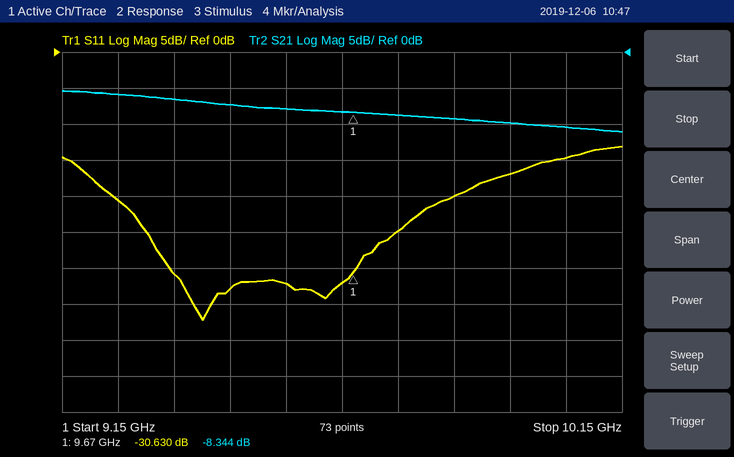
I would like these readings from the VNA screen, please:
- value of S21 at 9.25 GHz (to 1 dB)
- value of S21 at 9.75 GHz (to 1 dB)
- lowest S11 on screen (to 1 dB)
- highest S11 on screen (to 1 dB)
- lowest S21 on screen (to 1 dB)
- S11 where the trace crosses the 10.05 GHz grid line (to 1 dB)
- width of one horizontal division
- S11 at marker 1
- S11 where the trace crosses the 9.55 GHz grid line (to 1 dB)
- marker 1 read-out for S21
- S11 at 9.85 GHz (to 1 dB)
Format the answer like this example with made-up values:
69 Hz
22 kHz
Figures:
-6 dB
-9 dB
-37 dB
-13 dB
-11 dB
-15 dB
100 MHz
-30.630 dB
-32 dB
-8.344 dB
-20 dB
